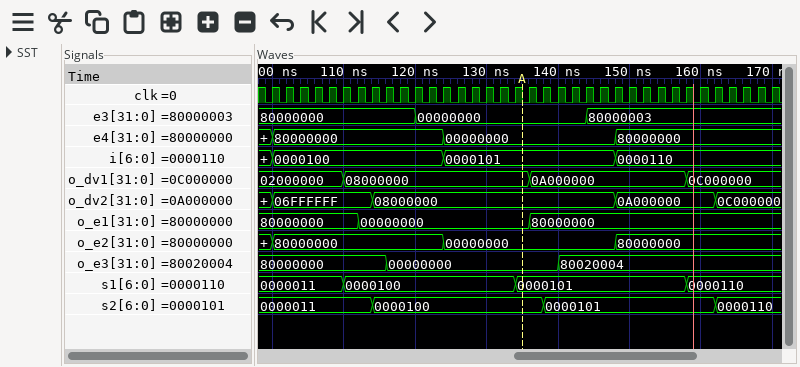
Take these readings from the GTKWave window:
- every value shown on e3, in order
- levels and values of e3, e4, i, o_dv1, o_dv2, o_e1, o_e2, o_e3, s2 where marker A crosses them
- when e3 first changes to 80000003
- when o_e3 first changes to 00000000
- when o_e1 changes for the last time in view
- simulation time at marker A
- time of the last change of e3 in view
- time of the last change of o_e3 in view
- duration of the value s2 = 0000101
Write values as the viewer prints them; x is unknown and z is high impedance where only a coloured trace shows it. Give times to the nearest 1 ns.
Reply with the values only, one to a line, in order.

80000000, 00000000, 80000003
e3=00000000, e4=00000000, i=0000101, o_dv1=08000000, o_dv2=08000000, o_e1=00000000, o_e2=00000000, o_e3=00000000, s2=0000100
144 ns
116 ns
136 ns
135 ns
144 ns
140 ns
24 ns
